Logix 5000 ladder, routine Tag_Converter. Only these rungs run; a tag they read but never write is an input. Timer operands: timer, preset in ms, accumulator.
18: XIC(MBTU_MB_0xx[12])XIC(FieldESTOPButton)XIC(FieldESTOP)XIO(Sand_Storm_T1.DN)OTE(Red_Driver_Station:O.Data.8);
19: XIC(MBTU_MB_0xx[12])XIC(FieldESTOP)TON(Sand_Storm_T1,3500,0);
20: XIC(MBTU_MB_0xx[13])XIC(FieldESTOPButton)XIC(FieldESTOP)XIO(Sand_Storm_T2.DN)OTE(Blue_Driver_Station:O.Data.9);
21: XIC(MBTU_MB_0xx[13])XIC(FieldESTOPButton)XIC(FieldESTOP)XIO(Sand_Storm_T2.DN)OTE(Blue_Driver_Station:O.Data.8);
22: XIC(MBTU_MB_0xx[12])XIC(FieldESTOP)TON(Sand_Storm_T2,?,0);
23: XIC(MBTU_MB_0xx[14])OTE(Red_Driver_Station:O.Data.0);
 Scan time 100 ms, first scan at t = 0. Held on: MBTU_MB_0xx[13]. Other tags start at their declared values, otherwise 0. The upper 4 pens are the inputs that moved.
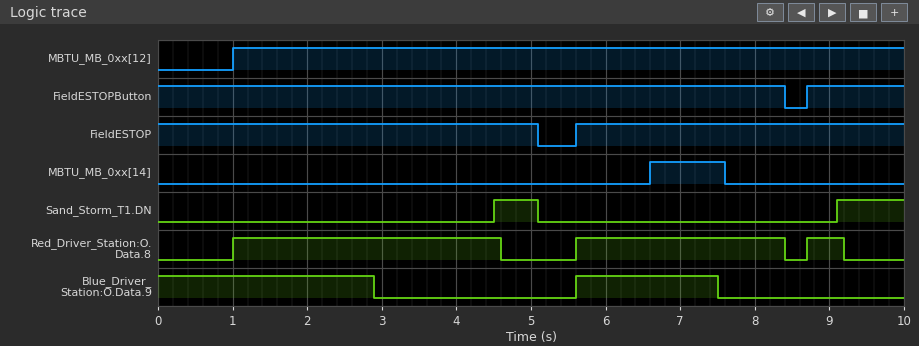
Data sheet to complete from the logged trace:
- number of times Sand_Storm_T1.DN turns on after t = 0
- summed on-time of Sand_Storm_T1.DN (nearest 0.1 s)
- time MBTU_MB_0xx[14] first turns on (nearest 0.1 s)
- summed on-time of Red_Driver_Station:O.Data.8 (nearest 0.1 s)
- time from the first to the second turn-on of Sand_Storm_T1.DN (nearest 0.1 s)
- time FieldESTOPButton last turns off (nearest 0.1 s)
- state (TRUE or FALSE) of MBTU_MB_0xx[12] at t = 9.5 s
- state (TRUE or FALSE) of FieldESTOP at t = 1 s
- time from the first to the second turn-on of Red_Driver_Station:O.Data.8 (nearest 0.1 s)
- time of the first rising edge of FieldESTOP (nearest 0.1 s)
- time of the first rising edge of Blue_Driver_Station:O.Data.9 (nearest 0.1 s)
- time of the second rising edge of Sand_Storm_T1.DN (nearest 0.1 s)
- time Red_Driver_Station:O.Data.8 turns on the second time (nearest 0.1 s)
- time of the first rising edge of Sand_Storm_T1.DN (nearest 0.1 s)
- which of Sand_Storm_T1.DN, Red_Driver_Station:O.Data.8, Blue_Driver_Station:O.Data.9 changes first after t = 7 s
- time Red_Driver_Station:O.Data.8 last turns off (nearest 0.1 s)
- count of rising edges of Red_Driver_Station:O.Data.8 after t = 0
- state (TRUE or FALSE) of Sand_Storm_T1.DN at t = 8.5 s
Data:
2
1.5 s
6.6 s
6.9 s
4.6 s
8.4 s
TRUE
TRUE
4.6 s
5.6 s
5.6 s
9.1 s
5.6 s
4.5 s
Blue_Driver_Station:O.Data.9
9.2 s
3
FALSE
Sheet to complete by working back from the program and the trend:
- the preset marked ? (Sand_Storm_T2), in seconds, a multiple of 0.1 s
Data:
1.8 s
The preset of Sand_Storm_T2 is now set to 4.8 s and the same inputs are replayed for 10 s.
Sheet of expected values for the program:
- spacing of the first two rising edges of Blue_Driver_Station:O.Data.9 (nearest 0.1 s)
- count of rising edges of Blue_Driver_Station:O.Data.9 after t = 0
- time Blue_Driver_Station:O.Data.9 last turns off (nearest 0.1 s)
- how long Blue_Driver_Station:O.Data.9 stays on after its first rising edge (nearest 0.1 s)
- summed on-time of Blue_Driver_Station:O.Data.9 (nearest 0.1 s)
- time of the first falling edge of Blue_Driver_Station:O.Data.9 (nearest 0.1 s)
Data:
3.1 s
2
8.4 s
2.8 s
9.2 s
5.1 s
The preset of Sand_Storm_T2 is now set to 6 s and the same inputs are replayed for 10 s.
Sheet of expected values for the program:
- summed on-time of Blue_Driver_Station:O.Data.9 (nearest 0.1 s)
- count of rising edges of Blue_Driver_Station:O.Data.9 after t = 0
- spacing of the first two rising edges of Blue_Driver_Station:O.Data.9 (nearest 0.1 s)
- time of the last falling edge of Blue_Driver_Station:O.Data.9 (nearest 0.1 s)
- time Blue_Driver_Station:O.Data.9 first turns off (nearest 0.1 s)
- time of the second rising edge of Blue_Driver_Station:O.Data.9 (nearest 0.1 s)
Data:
9.2 s
2
3.1 s
8.4 s
5.1 s
8.7 s
